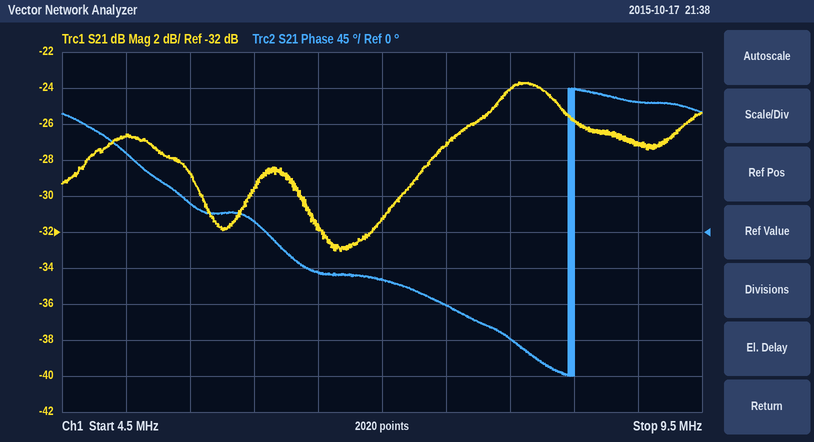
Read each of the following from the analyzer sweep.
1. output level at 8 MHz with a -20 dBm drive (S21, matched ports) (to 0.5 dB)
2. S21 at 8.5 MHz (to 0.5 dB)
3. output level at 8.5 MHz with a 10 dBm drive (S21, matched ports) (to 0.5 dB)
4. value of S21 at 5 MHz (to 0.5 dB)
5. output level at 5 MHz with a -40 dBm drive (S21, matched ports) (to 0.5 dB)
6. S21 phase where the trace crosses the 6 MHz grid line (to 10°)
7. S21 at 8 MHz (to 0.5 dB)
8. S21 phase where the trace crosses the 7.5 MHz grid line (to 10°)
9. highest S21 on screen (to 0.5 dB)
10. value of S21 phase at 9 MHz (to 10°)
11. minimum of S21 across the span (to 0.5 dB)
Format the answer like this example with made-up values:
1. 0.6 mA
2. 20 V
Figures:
1. -44.0 dBm
2. -26.0 dB
3. -16.0 dBm
4. -26.5 dB
5. -66.5 dBm
6. 10°
7. -24.0 dB
8. -90°
9. -23.5 dB
10. 160°
11. -33.0 dB
